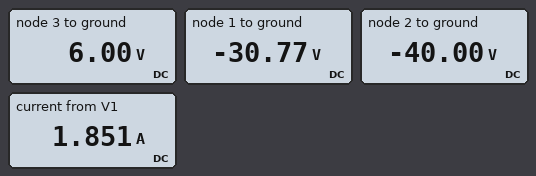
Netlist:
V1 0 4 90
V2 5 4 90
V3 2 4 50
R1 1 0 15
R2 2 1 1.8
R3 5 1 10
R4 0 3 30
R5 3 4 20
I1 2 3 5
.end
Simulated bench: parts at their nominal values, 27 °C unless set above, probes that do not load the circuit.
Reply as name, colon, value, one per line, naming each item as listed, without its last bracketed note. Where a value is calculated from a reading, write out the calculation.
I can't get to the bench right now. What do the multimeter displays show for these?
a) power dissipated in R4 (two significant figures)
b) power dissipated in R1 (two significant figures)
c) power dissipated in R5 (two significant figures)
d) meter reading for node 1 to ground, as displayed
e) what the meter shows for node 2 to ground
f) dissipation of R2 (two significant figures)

power dissipated in R4: (6 V)^2 / 30 Ω = 1.2 W
power dissipated in R1: (0 V - (-30.77 V))^2 / 15 Ω = 63 W
power dissipated in R5: (6 V - (-90 V))^2 / 20 Ω = 460 W
meter reading for node 1 to ground, as displayed: -30.77 V
what the meter shows for node 2 to ground: -40.00 V
dissipation of R2: (-30.77 V - (-40 V))^2 / 1.8 Ω = 47 W
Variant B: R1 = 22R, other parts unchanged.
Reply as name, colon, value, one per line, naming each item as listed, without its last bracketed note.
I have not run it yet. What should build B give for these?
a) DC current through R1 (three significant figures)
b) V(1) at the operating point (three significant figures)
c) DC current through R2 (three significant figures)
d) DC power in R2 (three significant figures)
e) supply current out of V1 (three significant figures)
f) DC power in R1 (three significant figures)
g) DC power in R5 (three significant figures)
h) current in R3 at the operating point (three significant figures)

DC current through R1: 1.44 A
V(1) at the operating point: -31.7 V
DC current through R2: 4.61 A
DC power in R2: 38.3 W
supply current out of V1: 1.24 A
DC power in R1: 45.7 W
DC power in R5: 461 W
current in R3 at the operating point: 3.17 A
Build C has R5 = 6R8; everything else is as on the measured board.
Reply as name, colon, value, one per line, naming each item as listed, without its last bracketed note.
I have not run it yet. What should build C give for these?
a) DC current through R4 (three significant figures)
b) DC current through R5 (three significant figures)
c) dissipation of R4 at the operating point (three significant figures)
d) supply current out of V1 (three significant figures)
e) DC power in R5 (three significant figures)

DC current through R4: 1.52 A
DC current through R5: 6.52 A
dissipation of R4 at the operating point: 69.5 W
supply current out of V1: 3.57 A
DC power in R5: 289 W
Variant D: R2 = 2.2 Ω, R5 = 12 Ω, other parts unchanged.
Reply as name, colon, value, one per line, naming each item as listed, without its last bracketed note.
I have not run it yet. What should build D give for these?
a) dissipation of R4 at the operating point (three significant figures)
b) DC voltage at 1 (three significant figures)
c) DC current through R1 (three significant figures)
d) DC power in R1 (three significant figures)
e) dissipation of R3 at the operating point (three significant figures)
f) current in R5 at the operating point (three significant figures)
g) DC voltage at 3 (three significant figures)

dissipation of R4 at the operating point: 15.3 W
DC voltage at 1: -29.3 V
DC current through R1: 1.95 A
DC power in R1: 57.1 W
dissipation of R3 at the operating point: 85.7 W
current in R5 at the operating point: 5.71 A
DC voltage at 3: -21.4 V
